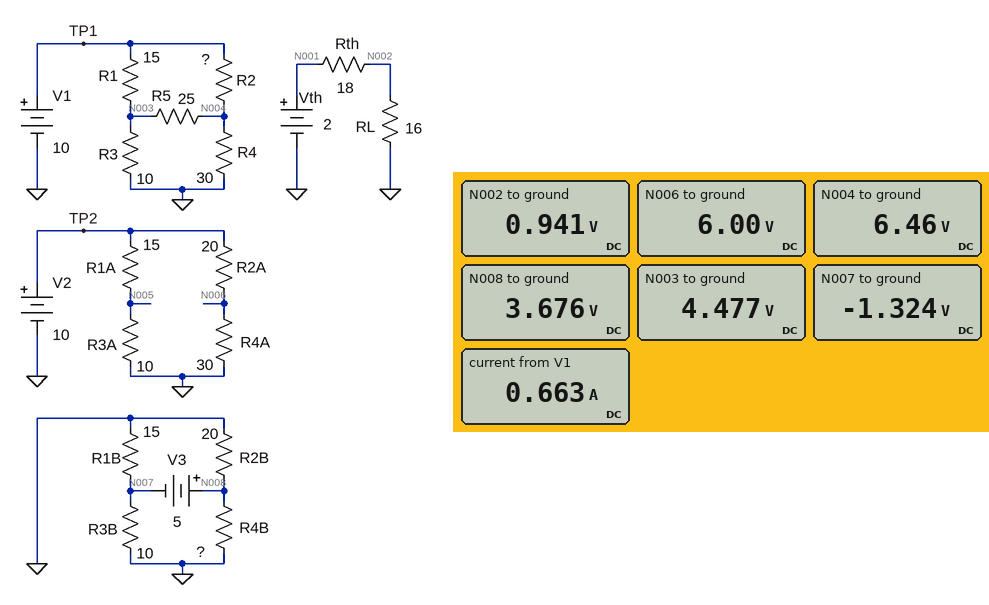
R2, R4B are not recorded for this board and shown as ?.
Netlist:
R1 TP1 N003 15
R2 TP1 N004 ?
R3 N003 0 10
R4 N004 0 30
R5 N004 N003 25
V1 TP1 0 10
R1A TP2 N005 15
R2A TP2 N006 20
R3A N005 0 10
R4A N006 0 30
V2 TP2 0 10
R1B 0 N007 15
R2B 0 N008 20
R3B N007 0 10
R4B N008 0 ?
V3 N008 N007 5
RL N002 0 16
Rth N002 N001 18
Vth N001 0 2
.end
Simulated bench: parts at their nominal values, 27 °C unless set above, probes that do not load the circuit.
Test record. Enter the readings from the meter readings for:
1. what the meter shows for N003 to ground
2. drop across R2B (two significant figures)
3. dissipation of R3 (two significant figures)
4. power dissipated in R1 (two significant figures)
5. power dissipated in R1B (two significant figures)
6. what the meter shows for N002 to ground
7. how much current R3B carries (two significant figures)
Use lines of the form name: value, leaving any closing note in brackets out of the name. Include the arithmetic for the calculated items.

what the meter shows for N003 to ground: 4.477 V
drop across R2B: 3.676 V = 3.7 V
dissipation of R3: (4.477 V)^2 / 10 Ω = 2.0 W
power dissipated in R1: (10 V - 4.477 V)^2 / 15 Ω = 2.0 W
power dissipated in R1B: (0 V - (-1.324 V))^2 / 15 Ω = 120 mW
what the meter shows for N002 to ground: 0.941 V
how much current R3B carries: (0 V - (-1.324 V)) / 10 Ω = 130 mA
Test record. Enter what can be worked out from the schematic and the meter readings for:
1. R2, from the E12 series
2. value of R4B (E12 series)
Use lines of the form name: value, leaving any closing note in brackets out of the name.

R2, from the E12 series: 12 Ω
value of R4B: 100 Ω
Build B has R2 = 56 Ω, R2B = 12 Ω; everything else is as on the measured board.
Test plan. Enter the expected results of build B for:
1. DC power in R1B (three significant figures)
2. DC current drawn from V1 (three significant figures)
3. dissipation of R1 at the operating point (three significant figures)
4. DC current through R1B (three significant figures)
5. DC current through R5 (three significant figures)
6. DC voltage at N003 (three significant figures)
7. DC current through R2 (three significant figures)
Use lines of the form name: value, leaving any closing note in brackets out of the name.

DC power in R1B: 215 mW
DC current drawn from V1: 517 mA
dissipation of R1 at the operating point: 2.45 W
DC current through R1B: 120 mA
DC current through R5: 10.1 mA
DC voltage at N003: 3.94 V
DC current through R2: 113 mA
